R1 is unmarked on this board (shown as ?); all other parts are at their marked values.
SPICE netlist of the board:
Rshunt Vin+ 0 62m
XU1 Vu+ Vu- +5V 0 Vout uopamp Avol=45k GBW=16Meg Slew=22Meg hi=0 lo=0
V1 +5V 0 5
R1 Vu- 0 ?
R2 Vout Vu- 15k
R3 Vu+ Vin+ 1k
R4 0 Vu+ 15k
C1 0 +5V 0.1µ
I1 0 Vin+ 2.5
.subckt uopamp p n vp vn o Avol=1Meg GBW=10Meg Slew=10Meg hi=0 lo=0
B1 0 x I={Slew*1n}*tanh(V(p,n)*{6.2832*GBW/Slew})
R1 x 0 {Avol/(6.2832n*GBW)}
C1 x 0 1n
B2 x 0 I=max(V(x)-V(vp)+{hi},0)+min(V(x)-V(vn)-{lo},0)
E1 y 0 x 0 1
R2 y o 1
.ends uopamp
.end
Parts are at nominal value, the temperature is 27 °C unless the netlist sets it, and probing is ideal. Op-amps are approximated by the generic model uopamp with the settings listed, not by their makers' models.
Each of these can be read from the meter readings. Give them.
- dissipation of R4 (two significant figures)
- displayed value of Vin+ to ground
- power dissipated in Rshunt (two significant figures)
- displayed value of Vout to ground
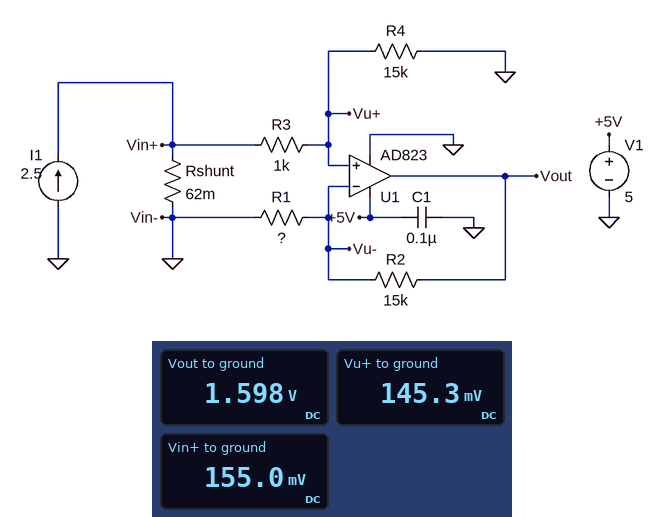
1.4 µW
155.0 mV
390 mW
1.598 V
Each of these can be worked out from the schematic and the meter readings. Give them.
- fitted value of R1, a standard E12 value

1.5 kΩ
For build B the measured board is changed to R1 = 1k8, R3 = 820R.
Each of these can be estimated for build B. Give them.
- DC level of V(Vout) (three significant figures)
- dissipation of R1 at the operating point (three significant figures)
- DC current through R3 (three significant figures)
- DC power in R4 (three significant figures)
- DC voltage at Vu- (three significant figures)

1.37 V
12.0 µW
9.80 µA
1.44 µW
147 mV
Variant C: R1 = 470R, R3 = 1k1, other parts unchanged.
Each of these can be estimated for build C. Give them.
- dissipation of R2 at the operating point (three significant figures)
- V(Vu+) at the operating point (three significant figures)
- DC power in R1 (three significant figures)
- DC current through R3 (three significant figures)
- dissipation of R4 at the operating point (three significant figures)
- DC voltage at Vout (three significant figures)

1.41 mW
144 mV
44.3 µW
9.63 µA
1.39 µW
4.75 V
